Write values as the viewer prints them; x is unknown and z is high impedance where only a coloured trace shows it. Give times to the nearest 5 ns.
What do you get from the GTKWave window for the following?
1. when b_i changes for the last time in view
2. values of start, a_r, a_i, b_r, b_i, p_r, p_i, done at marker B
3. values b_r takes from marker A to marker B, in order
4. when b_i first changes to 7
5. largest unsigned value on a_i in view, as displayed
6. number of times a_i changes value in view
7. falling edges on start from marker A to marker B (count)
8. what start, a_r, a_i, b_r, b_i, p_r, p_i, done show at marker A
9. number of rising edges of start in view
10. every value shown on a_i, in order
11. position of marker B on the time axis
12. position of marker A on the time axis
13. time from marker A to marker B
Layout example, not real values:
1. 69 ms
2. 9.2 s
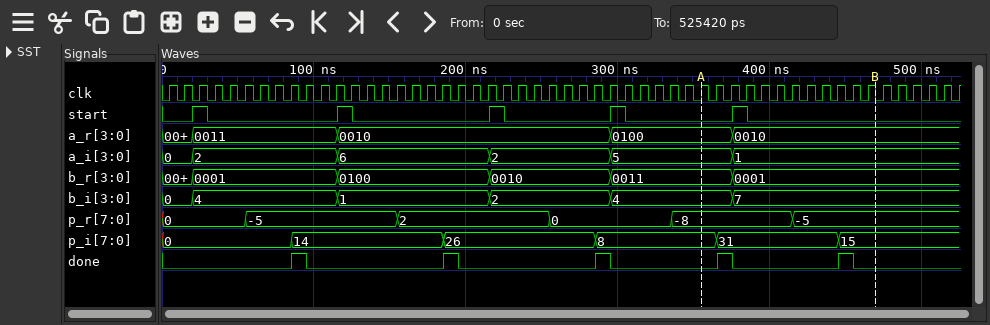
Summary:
1. 375 ns
2. start=0, a_r=0010, a_i=1, b_r=0001, b_i=7, p_r=-5, p_i=15, done=0
3. 0011, 0001
4. 375 ns
5. 6
6. 5
7. 1
8. start=0, a_r=0100, a_i=5, b_r=0011, b_i=4, p_r=-8, p_i=8, done=0
9. 5
10. 0, 2, 6, 2, 5, 1
11. 470 ns
12. 355 ns
13. 115 ns
